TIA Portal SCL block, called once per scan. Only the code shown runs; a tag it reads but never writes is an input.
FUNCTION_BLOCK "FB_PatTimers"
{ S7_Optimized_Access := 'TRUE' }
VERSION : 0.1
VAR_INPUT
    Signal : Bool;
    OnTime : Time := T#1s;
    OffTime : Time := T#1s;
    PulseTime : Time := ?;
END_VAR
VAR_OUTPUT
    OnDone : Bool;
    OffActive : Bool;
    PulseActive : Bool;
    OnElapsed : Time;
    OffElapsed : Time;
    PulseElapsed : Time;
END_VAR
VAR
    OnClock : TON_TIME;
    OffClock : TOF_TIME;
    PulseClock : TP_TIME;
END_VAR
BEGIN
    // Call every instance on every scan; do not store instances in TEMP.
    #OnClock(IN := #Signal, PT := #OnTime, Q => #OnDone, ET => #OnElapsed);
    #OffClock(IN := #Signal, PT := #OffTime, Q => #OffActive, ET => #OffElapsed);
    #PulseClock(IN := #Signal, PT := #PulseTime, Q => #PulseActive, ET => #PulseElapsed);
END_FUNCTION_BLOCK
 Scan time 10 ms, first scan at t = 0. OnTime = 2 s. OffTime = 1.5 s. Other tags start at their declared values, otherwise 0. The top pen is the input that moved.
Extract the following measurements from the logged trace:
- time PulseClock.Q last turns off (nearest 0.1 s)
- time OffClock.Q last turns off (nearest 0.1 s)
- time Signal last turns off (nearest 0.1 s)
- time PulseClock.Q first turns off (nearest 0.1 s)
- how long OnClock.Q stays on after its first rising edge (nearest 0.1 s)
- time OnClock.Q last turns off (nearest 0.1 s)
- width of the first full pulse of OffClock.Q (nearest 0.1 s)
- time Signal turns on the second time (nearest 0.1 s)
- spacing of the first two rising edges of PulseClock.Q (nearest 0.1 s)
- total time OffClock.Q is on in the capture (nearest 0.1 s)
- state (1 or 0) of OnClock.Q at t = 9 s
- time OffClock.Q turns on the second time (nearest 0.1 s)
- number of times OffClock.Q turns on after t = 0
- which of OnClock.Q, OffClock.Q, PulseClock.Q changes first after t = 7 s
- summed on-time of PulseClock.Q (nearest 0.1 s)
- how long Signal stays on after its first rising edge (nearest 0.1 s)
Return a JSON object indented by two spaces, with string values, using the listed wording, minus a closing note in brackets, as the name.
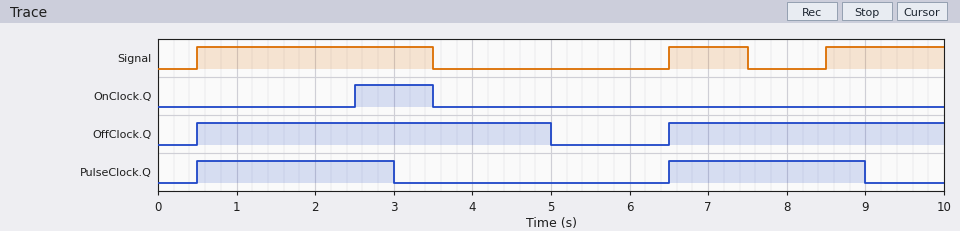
{
  "time PulseClock.Q last turns off": "9.0 s",
  "time OffClock.Q last turns off": "5.0 s",
  "time Signal last turns off": "7.5 s",
  "time PulseClock.Q first turns off": "3.0 s",
  "how long OnClock.Q stays on after its first rising edge": "1.0 s",
  "time OnClock.Q last turns off": "3.5 s",
  "width of the first full pulse of OffClock.Q": "4.5 s",
  "time Signal turns on the second time": "6.5 s",
  "spacing of the first two rising edges of PulseClock.Q": "6.0 s",
  "total time OffClock.Q is on in the capture": "8.0 s",
  "state (1 or 0) of OnClock.Q at t = 9 s": "0",
  "time OffClock.Q turns on the second time": "6.5 s",
  "number of times OffClock.Q turns on after t = 0": "2",
  "which of OnClock.Q, OffClock.Q, PulseClock.Q changes first after t = 7 s": "PulseClock.Q",
  "summed on-time of PulseClock.Q": "5.0 s",
  "how long Signal stays on after its first rising edge": "3.0 s"
}
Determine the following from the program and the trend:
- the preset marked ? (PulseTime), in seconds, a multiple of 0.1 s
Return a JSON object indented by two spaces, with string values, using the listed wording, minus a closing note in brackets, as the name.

{
  "the preset marked ? (PulseTime), in seconds, a multiple of 0.1 s": "2.5 s"
}
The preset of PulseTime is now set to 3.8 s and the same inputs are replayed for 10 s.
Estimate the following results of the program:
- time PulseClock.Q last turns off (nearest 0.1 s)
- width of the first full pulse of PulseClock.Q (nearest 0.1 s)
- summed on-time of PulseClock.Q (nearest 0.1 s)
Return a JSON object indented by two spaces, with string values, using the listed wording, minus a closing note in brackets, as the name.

{
  "time PulseClock.Q last turns off": "4.3 s",
  "width of the first full pulse of PulseClock.Q": "3.8 s",
  "summed on-time of PulseClock.Q": "7.3 s"
}
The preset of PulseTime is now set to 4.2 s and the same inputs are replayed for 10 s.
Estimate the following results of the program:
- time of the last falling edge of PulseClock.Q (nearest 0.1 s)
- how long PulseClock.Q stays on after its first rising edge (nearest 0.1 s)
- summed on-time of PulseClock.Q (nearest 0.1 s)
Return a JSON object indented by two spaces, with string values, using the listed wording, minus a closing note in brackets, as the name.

{
  "time of the last falling edge of PulseClock.Q": "4.7 s",
  "how long PulseClock.Q stays on after its first rising edge": "4.2 s",
  "summed on-time of PulseClock.Q": "7.7 s"
}
